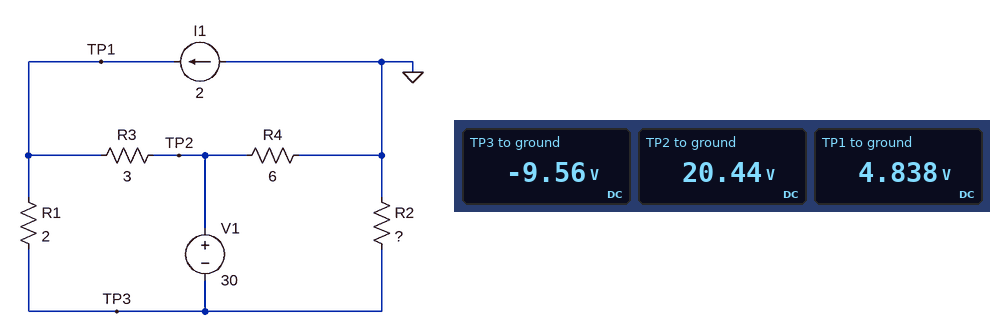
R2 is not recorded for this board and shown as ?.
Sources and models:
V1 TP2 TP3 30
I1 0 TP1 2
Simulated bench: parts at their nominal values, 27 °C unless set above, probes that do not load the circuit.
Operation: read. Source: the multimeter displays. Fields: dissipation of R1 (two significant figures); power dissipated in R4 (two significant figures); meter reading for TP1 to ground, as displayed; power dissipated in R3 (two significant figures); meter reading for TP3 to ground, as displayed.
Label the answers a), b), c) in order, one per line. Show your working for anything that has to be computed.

a) (4.838 V - (-9.56 V))^2 / 2 Ω = 100 W
b) (20.44 V)^2 / 6 Ω = 70 W
c) 4.838 V
d) (20.44 V - 4.838 V)^2 / 3 Ω = 81 W
e) -9.56 V
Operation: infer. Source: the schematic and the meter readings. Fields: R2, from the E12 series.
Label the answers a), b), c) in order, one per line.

a) 6.8 Ω
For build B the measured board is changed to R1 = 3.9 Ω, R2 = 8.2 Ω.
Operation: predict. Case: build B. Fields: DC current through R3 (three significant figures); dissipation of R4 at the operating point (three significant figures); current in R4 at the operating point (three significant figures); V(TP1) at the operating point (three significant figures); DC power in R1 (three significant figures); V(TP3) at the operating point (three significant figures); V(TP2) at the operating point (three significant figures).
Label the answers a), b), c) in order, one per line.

a) 3.22 A
b) 64.1 W
c) 3.27 A
d) 9.95 V
e) 106 W
f) -10.4 V
g) 19.6 V
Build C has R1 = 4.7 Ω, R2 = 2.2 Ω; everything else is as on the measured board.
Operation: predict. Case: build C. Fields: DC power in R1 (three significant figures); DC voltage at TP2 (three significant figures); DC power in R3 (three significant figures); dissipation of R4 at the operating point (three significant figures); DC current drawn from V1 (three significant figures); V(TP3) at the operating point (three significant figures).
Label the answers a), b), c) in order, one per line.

a) 103 W
b) 25.2 V
c) 21.5 W
d) 106 W
e) 6.87 A
f) -4.83 V
